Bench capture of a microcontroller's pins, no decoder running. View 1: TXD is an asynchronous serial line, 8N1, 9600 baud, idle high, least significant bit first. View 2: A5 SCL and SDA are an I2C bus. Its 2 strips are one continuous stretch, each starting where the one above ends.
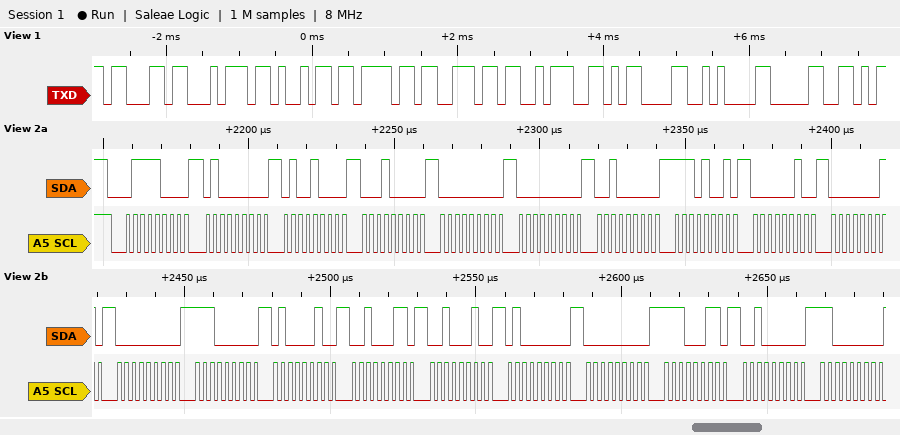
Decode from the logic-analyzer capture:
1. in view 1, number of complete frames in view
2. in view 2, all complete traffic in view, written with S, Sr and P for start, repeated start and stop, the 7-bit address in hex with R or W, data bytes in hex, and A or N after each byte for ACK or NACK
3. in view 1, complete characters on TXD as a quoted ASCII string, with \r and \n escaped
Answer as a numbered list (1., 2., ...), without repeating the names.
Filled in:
1. 9
2. S 3CW A 40 A 48 A 10 A 00 A 00 A 20 A E9 A 02 A 01 A 00 A E0 A 42 A 23 A 22 A 40 A 00 A E3 A 20 A C0 A
3. "ction:\r\n0"
